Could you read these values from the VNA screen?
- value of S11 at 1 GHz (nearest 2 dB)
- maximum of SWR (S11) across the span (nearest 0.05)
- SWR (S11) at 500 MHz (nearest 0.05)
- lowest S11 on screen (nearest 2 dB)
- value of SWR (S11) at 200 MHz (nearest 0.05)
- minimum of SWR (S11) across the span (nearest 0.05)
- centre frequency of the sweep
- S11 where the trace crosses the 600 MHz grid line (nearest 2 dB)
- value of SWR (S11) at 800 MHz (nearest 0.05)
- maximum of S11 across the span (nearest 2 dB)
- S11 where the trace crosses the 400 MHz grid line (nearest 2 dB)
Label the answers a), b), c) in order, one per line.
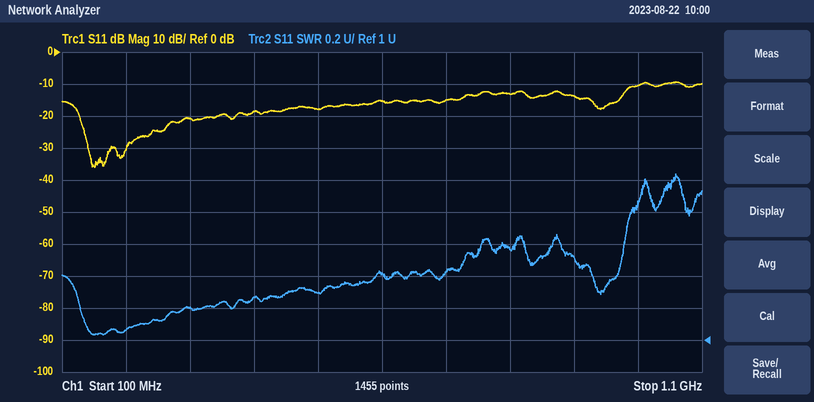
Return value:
a) -10 dB
b) 2.05
c) 1.30
d) -36 dB
e) 1.05
f) 1.05
g) 600 MHz
h) -16 dB
i) 1.55
j) -10 dB
k) -18 dB
